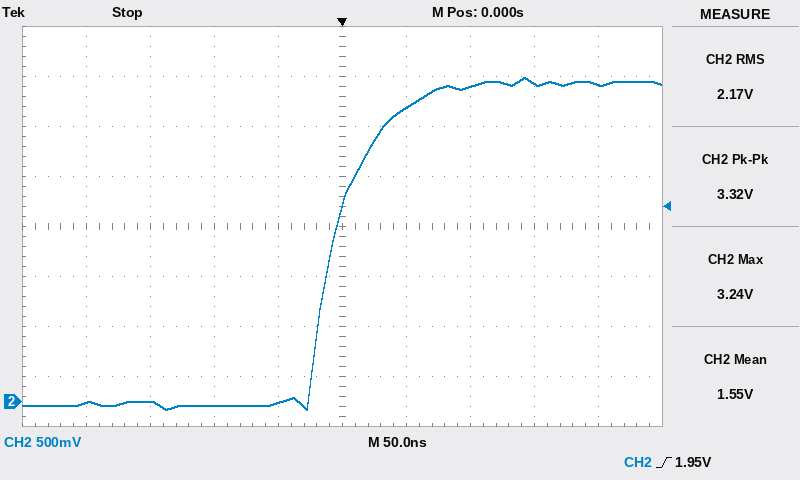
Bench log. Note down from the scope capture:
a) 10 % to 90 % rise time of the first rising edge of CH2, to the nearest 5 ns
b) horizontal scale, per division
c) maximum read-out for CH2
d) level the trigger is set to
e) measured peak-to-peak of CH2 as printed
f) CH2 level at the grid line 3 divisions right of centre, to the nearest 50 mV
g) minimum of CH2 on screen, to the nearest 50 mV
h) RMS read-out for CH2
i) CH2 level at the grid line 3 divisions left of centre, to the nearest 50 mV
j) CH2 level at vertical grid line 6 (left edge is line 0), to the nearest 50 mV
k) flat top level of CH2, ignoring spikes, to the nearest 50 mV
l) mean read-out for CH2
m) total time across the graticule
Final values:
65 ns
50 ns
3.24 V
1.95 V
3.32 V
3.20 V
-100 mV
2.17 V
0 mV
2.95 V
3.20 V
1.55 V
500 ns
